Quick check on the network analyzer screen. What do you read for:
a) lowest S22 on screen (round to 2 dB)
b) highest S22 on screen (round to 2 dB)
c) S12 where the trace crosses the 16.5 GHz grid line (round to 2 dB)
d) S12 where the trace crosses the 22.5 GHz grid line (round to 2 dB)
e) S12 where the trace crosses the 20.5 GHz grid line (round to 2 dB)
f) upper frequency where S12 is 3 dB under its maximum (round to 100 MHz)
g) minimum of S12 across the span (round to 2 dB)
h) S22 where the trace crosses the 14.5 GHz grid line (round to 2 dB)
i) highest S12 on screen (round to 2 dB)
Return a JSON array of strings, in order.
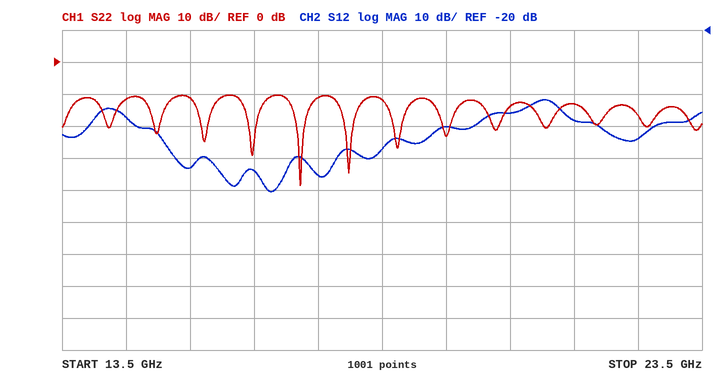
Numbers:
["-38 dB", "-10 dB", "-64 dB", "-54 dB", "-46 dB", "21.3 GHz", "-70 dB", "-12 dB", "-42 dB"]
